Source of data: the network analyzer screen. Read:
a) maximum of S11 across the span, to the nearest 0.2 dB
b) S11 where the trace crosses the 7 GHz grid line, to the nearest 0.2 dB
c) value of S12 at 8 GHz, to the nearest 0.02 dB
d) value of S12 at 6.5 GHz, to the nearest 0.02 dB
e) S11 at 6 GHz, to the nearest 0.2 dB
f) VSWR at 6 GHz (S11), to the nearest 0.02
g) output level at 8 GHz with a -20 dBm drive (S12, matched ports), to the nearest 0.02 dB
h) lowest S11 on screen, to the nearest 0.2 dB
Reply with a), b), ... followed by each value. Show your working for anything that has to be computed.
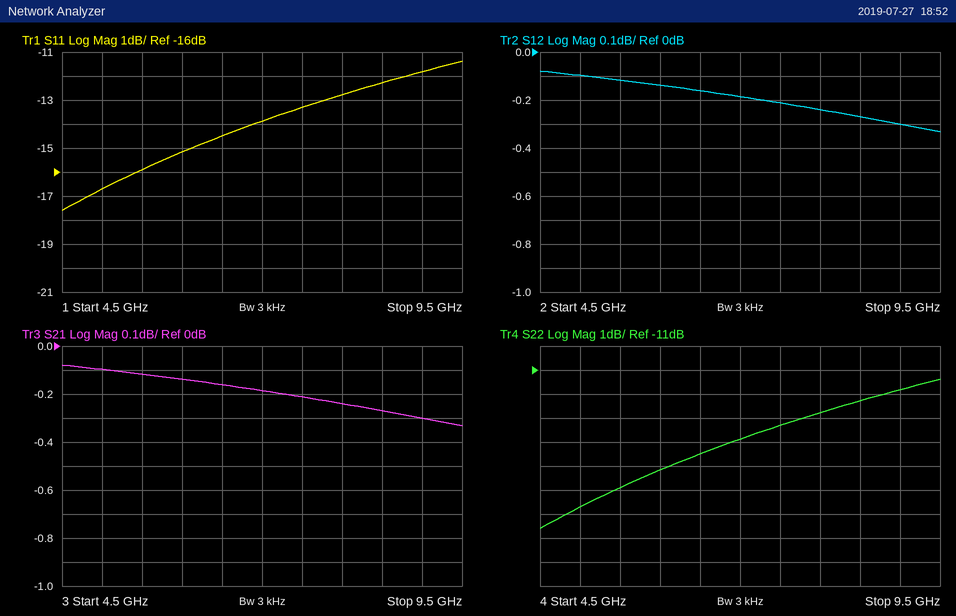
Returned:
a) -11.4 dB
b) -13.8 dB
c) -0.24 dB
d) -0.16 dB
e) -15.2 dB
f) |Γ| = 10^(-15.2/20) = 0.1738; VSWR = (1 + 0.1738)/(1 − 0.1738) ≈ 1.42
g) -20 dBm + (-0.24 dB) = -20.24 dBm
h) -17.6 dB
